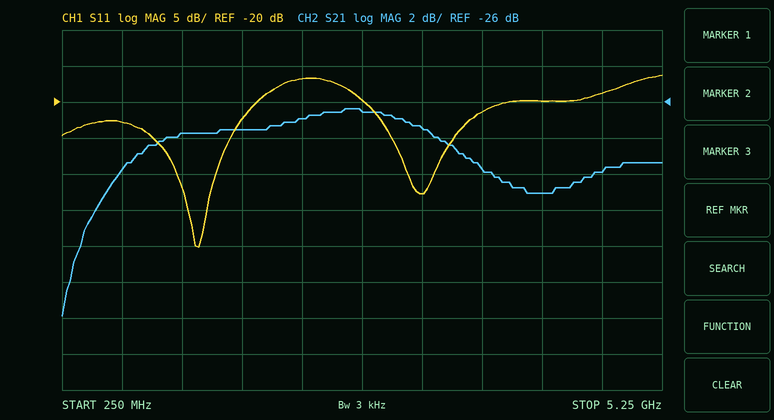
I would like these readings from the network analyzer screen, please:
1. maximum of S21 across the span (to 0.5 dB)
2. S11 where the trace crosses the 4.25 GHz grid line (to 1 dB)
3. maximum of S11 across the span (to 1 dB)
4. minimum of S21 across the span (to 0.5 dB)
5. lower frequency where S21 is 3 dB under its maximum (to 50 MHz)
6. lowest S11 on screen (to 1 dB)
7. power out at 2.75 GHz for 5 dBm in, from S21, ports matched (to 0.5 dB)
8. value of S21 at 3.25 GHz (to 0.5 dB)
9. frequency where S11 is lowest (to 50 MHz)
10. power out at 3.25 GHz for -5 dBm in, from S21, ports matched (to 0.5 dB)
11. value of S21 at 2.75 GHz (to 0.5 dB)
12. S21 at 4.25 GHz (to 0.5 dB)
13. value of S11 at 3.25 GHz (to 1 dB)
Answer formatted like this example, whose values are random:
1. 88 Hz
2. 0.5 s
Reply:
1. -26.5 dB
2. -20 dB
3. -16 dB
4. -38.0 dB
5. 800 MHz
6. -40 dB
7. -21.5 dBm
8. -27.5 dB
9. 1.40 GHz
10. -32.5 dBm
11. -26.5 dB
12. -31.0 dB
13. -33 dB
